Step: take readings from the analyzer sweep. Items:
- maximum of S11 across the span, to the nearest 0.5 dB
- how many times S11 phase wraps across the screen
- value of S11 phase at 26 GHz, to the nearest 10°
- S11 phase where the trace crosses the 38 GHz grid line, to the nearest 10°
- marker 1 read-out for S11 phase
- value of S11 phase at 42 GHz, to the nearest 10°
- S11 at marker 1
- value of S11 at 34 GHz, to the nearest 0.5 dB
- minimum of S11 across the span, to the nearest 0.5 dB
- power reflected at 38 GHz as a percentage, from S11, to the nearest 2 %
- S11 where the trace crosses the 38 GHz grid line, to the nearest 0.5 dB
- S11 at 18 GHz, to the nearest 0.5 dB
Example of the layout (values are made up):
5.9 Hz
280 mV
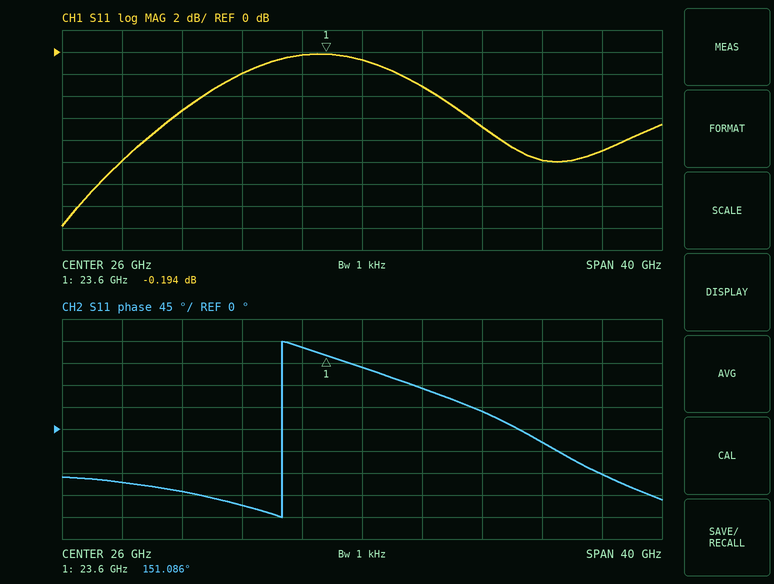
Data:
0.0 dB
1
130°
-30°
151.086°
-90°
-0.194 dB
-7.0 dB
-16.0 dB
10 %
-10.0 dB
-2.0 dB
